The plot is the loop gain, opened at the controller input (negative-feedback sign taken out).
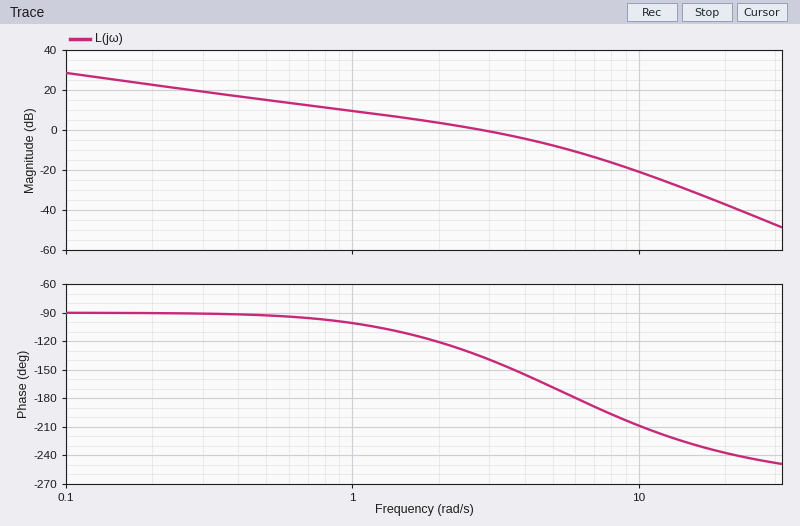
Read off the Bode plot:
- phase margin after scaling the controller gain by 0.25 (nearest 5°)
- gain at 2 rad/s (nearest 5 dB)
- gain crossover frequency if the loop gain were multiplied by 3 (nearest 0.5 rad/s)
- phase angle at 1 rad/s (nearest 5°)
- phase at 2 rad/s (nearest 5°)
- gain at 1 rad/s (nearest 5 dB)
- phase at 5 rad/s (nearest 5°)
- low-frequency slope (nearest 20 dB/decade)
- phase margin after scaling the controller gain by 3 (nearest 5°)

85°
5 dB
5.5 rad/s
-100°
-120°
10 dB
-170°
-20 dB/decade
5°
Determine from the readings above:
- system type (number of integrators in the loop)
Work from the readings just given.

1
